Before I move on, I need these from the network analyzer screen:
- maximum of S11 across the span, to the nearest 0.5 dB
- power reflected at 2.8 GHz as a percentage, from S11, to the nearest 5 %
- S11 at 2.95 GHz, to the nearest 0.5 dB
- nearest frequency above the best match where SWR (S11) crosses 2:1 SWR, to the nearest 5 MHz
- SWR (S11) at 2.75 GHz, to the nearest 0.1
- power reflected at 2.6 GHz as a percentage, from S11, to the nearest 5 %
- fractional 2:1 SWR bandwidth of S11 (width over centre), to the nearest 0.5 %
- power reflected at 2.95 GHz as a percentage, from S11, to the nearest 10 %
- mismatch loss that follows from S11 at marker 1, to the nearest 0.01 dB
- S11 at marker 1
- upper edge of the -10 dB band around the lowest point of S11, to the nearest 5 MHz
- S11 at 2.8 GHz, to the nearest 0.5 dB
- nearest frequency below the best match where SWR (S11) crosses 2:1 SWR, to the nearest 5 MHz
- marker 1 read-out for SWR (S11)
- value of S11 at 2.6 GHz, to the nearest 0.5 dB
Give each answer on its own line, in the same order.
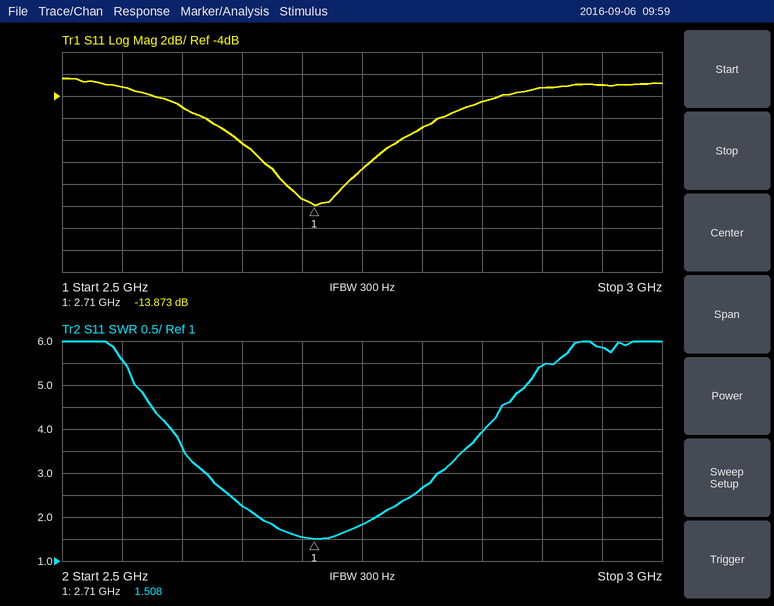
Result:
-2.5 dB
20 %
-3.0 dB
2.760 GHz
1.8
30 %
3.5 %
50 %
0.18 dB
-13.873 dB
2.755 GHz
-7.0 dB
2.665 GHz
1.508
-5.0 dB
